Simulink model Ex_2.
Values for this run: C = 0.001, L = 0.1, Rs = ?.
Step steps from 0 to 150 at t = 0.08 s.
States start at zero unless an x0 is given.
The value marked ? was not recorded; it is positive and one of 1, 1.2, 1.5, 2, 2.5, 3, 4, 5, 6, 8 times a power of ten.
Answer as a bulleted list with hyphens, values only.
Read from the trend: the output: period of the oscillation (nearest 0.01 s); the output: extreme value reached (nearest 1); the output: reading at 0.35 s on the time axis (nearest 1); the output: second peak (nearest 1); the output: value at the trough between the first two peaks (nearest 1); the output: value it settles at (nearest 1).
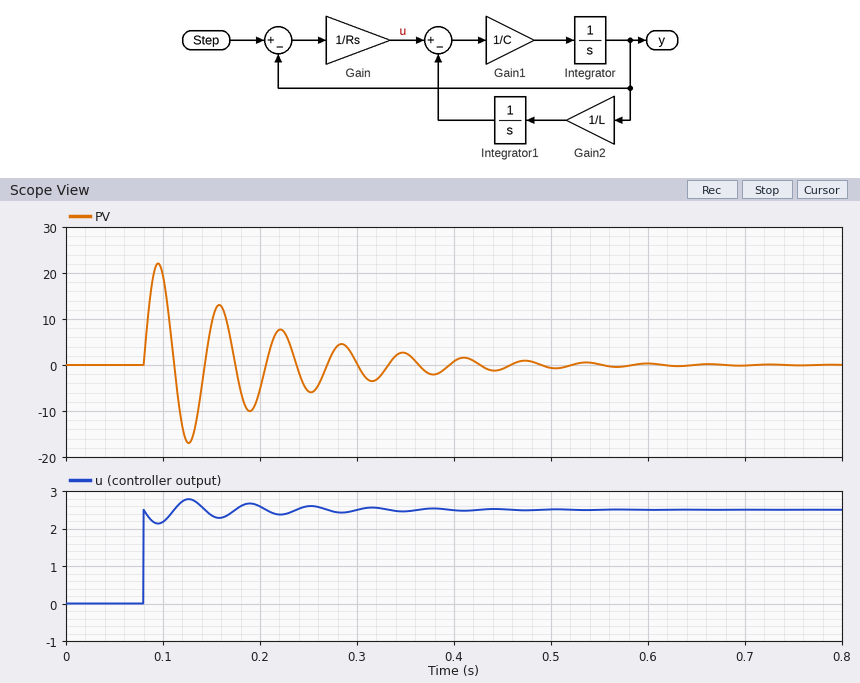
- 0.06 s
- 22
- 3
- 13
- -17
- 0
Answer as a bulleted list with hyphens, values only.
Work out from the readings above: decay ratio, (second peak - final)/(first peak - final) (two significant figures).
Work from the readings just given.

- 0.59
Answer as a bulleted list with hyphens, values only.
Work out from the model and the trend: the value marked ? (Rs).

- 60
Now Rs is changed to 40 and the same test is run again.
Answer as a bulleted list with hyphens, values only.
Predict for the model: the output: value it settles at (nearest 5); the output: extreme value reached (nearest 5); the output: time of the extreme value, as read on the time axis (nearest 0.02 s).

- 0
- 30
- 0.10 s
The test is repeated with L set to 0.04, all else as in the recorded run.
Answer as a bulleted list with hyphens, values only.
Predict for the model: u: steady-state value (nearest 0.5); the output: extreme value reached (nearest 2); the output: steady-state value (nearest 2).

- 2.5
- 14
- 0
